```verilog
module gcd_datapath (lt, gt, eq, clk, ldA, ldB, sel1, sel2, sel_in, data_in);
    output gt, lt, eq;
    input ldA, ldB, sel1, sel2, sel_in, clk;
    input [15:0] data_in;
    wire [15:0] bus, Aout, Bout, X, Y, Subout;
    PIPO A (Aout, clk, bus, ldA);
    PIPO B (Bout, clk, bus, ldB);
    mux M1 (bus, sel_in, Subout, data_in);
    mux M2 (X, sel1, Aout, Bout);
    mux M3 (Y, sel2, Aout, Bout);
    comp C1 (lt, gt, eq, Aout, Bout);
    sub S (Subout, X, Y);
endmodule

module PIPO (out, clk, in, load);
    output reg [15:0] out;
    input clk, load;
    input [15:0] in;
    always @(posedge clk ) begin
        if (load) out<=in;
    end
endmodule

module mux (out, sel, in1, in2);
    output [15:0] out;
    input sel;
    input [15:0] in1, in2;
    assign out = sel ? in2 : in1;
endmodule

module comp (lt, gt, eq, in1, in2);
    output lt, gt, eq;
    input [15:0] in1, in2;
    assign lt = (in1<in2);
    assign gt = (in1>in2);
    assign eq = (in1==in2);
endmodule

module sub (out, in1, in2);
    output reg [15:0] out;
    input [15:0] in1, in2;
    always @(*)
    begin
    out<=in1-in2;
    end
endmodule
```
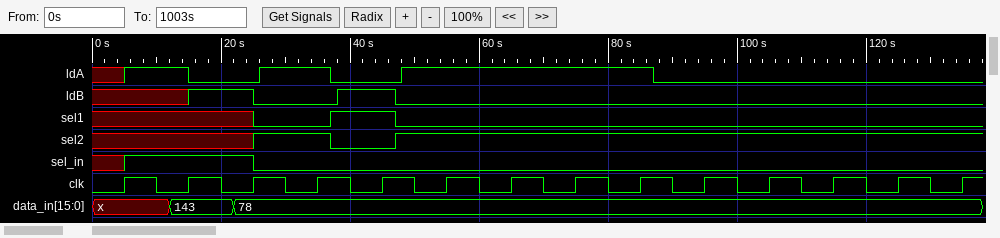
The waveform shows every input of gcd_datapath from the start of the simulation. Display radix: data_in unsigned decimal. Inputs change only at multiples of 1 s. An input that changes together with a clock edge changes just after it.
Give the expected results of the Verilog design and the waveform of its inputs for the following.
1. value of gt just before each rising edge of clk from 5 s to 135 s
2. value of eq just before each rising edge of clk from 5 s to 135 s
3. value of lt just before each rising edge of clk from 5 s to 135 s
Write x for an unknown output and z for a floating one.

x x x 1 0 1 1 1 1 0 0 0 0 0
x x x 0 0 0 0 0 0 1 1 1 1 1
x x x 0 1 0 0 0 0 0 0 0 0 0
